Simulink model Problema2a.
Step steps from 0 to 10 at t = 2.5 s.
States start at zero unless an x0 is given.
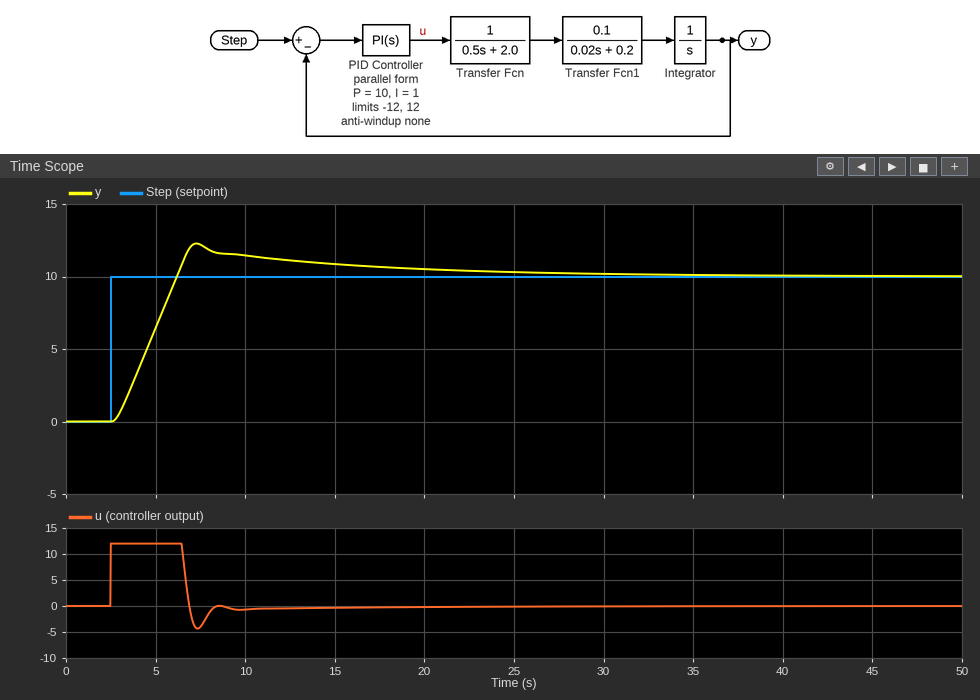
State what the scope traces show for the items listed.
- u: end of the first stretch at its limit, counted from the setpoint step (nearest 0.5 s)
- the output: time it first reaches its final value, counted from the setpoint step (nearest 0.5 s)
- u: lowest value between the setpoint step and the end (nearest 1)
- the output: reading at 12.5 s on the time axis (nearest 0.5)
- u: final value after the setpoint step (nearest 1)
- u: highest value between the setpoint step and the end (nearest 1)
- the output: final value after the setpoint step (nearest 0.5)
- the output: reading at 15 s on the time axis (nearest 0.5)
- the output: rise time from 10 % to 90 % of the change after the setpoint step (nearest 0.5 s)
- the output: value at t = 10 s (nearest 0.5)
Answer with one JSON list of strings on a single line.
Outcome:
["4.0 s", "3.5 s", "-4", "11.0", "0", "12", "10.0", "11.0", "2.5 s", "11.5"]
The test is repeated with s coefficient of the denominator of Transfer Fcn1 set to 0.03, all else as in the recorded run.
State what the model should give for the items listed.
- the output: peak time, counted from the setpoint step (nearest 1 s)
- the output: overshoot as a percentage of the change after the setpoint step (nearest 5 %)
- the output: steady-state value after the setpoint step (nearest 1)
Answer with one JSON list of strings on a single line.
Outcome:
["5 s", "25 %", "10"]
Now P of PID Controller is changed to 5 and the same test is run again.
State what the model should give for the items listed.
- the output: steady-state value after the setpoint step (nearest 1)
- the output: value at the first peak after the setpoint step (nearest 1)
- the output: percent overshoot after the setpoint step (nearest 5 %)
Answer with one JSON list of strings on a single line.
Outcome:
["10", "14", "35 %"]
